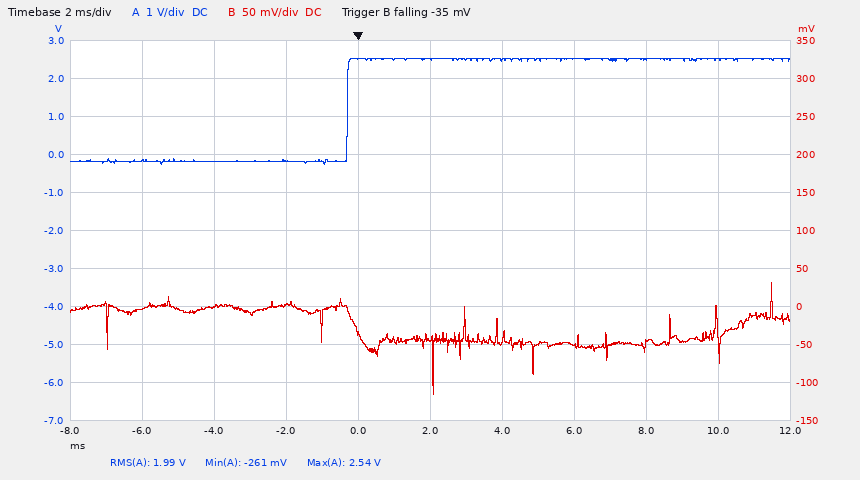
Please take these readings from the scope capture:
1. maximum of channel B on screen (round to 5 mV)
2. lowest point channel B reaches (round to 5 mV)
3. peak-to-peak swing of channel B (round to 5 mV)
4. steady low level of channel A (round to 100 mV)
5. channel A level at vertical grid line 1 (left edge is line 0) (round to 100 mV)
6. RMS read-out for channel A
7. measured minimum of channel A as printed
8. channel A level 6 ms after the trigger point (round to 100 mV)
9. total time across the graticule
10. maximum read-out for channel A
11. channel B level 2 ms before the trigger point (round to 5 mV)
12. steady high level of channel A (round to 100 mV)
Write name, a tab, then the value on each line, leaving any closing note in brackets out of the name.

maximum of channel B on screen	30 mV
lowest point channel B reaches	-115 mV
peak-to-peak swing of channel B	145 mV
steady low level of channel A	-200 mV
channel A level at vertical grid line 1 (left edge is line 0)	-200 mV
RMS read-out for channel A	1.99 V
measured minimum of channel A as printed	-261 mV
channel A level 6 ms after the trigger point	2.5 V
total time across the graticule	20 ms
maximum read-out for channel A	2.54 V
channel B level 2 ms before the trigger point	0 mV
steady high level of channel A	2.5 V
